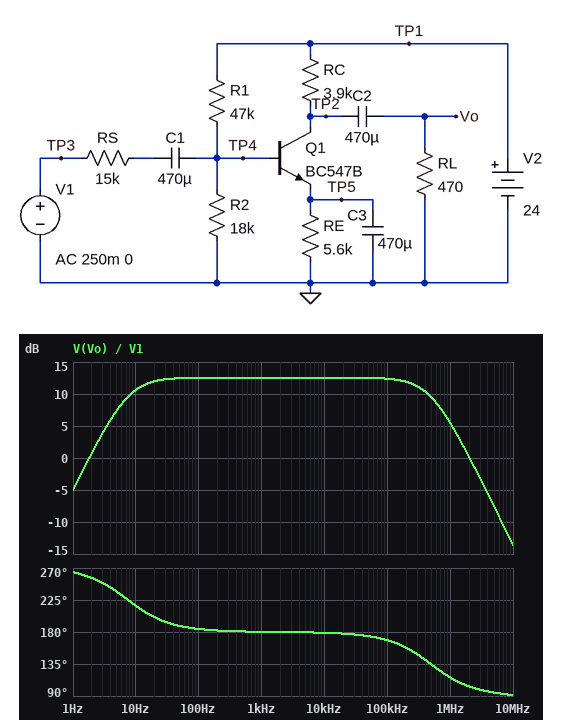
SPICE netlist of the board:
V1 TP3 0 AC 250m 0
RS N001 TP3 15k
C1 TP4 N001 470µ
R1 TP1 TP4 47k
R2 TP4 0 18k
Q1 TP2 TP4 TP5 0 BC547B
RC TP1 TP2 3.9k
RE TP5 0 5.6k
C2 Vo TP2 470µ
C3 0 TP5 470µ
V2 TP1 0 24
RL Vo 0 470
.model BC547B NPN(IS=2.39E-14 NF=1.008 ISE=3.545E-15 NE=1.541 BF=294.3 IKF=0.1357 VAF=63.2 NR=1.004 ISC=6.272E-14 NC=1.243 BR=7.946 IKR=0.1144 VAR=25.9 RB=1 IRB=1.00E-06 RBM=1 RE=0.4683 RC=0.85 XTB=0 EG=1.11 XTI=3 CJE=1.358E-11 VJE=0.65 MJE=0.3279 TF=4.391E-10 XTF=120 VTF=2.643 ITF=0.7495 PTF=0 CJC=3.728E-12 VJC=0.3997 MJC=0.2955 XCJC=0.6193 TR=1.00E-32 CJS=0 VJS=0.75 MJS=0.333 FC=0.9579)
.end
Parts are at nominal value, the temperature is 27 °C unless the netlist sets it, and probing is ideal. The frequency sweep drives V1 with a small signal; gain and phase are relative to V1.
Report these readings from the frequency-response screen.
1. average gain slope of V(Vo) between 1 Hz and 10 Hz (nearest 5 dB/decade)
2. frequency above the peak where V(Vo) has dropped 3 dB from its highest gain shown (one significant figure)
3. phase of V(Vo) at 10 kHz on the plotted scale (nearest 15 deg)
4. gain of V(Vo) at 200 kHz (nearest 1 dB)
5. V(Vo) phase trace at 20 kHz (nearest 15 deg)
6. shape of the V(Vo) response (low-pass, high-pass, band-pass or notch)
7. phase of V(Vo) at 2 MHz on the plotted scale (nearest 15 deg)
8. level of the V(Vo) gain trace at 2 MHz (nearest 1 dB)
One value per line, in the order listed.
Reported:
15 dB/decade
500 kHz
180 deg
12 dB
180 deg
band-pass
105 deg
0 dB
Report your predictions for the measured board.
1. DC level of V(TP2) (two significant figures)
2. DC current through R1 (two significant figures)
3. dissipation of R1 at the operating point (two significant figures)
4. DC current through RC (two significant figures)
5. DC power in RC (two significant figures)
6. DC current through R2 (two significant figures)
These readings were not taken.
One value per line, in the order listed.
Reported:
20 V
370 µA
6.4 mW
1.1 mA
4.4 mW
370 µA
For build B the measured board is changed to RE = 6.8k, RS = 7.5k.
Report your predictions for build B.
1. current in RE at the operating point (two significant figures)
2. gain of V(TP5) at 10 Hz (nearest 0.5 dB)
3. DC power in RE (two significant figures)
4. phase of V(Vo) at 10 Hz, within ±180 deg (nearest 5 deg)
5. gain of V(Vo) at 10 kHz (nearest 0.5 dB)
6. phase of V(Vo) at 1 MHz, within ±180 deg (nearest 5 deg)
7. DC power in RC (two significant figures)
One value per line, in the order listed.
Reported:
880 µA
-8.5 dB
5.3 mW
-140 deg
15.5 dB
125 deg
3.0 mW
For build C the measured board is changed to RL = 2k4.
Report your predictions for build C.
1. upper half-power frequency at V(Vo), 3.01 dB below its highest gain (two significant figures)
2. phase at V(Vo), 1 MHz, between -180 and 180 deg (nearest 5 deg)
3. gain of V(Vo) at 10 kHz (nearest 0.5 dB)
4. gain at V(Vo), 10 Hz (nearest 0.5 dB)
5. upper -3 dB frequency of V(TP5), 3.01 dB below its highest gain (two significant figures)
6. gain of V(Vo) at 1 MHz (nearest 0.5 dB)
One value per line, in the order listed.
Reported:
300 kHz
105 deg
23.5 dB
21.5 dB
7.4 Hz
12.5 dB
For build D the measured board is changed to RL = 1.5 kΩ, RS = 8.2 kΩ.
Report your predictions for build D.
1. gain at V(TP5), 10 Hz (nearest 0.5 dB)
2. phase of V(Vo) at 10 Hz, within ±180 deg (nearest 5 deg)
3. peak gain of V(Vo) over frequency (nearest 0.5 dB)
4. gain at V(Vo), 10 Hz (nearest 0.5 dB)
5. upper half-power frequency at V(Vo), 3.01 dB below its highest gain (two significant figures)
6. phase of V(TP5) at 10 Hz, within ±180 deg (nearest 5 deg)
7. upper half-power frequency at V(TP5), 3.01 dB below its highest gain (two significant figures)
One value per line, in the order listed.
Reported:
-8.0 dB
-140 deg
24.5 dB
22.0 dB
430 kHz
-50 deg
8.5 Hz
